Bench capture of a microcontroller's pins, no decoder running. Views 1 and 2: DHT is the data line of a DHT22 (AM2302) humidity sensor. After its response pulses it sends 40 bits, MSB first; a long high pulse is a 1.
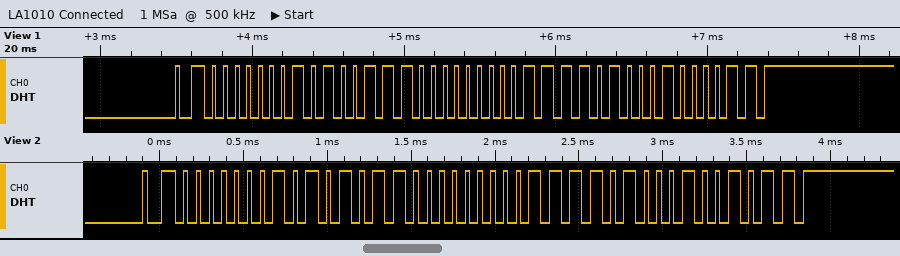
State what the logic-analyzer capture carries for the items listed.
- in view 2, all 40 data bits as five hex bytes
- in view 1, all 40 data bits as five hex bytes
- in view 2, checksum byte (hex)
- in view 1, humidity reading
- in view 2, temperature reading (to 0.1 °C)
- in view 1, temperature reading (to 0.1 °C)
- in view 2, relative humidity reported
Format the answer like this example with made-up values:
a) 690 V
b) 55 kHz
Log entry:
a) 01 56 00 F4 4B
b) 01 4E 00 F4 43
c) 0x4B
d) 33.4 %
e) 24.4 °C
f) 24.4 °C
g) 34.2 %
